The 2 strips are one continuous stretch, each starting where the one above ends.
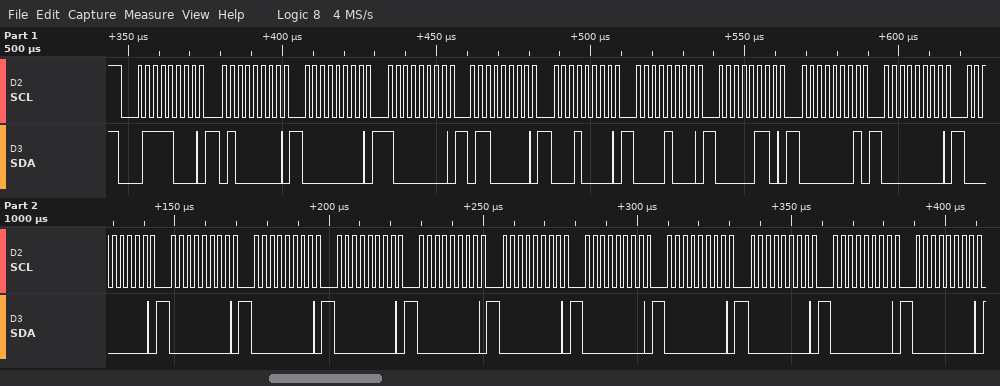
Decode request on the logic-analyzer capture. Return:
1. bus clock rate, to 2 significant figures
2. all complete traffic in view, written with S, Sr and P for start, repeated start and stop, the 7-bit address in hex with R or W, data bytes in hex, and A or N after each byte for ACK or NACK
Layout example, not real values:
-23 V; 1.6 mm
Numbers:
400 kHz; S 3CW A 40 A 00 A 80 A 60 A 10 A 08 A 06 A 01 A 00 A 00 A 00 A 00 A 00 A 00 A 00 A 00 A 00 A 00 A 00 A 00 A
